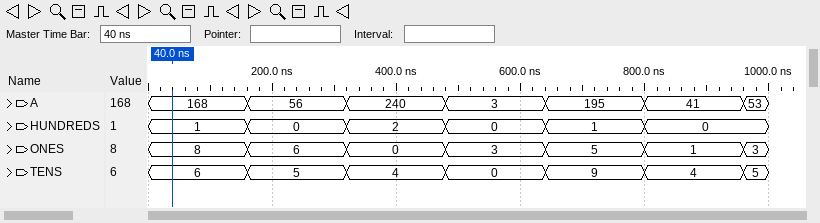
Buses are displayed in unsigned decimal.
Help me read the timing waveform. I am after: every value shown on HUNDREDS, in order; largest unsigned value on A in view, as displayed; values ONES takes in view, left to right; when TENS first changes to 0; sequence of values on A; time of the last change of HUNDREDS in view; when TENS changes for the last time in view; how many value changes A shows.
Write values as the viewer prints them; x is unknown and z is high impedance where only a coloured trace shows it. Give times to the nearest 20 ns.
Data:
1, 0, 2, 0, 1, 0
240
8, 6, 0, 3, 5, 1, 3
480 ns
168, 56, 240, 3, 195, 41, 53
800 ns
960 ns
6
